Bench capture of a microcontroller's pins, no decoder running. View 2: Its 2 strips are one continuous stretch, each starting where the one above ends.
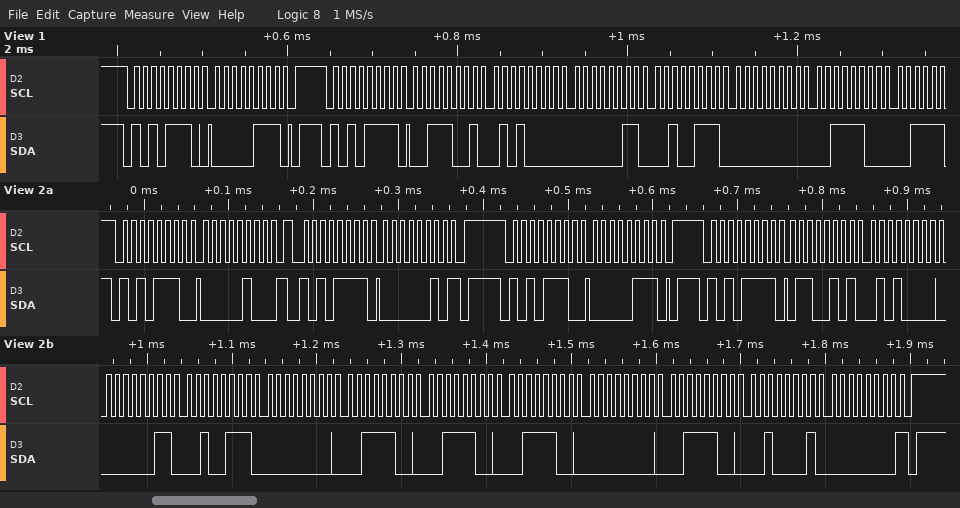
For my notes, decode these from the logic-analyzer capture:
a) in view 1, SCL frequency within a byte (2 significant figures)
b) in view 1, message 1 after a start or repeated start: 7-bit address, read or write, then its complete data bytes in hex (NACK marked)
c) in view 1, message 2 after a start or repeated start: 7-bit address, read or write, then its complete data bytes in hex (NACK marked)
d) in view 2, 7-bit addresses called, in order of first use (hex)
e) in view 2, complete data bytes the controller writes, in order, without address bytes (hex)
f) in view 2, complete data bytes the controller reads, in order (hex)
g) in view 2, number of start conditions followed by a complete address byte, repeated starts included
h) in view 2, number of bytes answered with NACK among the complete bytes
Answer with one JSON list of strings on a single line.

["100 kHz", "0x57 write: 07", "0x57 read: 39 50 03 27 00 3C", "0x57", "04 07", "02 65 50 03 27 00 3C 3C 3C 00 3C 21 00", "4", "2"]
